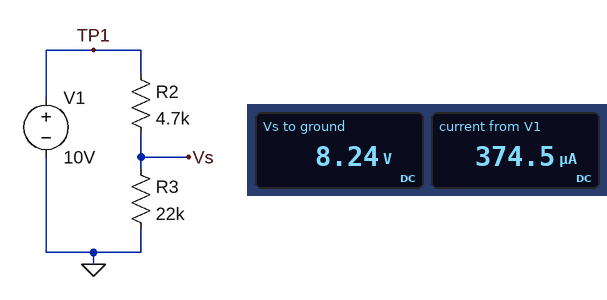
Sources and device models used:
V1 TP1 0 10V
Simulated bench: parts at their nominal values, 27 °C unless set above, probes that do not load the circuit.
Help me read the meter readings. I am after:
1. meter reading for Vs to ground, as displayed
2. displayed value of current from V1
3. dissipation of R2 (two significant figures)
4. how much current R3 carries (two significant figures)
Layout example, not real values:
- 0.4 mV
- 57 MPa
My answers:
- 8.24 V
- 374.5 µA
- 660 µW
- 370 µA
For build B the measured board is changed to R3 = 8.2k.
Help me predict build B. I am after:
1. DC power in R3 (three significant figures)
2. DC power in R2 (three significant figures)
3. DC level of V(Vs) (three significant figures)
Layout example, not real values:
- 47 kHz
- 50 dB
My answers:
- 4.93 mW
- 2.82 mW
- 6.36 V
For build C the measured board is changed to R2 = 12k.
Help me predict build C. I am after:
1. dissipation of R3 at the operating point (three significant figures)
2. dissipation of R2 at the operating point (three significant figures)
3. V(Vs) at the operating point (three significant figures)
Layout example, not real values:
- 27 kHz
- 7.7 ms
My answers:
- 1.90 mW
- 1.04 mW
- 6.47 V
